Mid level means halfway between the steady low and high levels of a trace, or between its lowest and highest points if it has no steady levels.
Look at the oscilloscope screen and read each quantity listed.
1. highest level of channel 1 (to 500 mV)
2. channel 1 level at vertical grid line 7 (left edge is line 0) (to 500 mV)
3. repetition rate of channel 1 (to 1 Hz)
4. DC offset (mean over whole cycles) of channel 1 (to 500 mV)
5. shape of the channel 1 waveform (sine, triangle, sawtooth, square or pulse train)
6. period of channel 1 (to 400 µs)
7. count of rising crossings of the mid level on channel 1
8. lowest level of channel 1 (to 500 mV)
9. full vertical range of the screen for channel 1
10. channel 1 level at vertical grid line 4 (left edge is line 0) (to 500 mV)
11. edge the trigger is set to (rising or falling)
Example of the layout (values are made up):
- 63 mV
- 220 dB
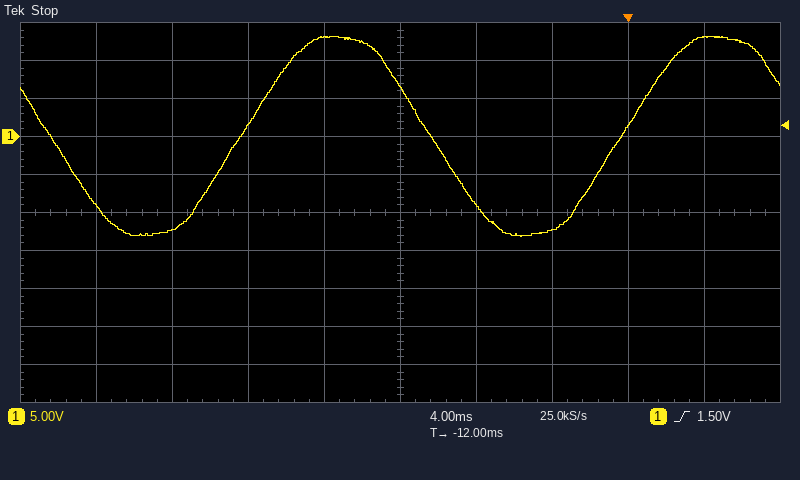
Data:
- 13.0 V
- -12.5 V
- 50 Hz
- 0.0 V
- sine
- 20.0 ms
- 2
- -13.0 V
- 50 V
- 13.0 V
- rising
